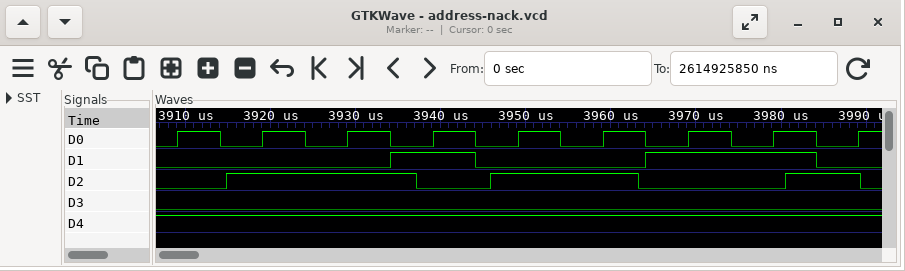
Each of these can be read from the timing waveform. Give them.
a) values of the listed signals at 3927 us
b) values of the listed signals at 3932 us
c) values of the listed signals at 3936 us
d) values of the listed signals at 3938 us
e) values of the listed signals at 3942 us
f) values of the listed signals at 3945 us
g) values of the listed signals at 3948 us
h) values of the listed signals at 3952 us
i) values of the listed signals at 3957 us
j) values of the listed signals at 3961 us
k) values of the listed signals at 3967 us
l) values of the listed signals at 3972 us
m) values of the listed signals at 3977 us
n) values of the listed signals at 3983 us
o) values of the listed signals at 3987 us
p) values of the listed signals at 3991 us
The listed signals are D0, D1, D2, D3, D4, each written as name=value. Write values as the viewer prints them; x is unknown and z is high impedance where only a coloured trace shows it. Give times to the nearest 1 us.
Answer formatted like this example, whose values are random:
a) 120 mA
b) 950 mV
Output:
a) D0=0, D1=0, D2=1, D3=0, D4=1
b) D0=1, D1=0, D2=1, D3=0, D4=1
c) D0=0, D1=1, D2=1, D3=0, D4=1
d) D0=0, D1=1, D2=0, D3=0, D4=1
e) D0=1, D1=1, D2=0, D3=0, D4=1
f) D0=0, D1=0, D2=0, D3=0, D4=1
g) D0=0, D1=0, D2=1, D3=0, D4=1
h) D0=1, D1=0, D2=1, D3=0, D4=1
i) D0=0, D1=0, D2=1, D3=0, D4=1
j) D0=1, D1=0, D2=1, D3=0, D4=1
k) D0=0, D1=1, D2=0, D3=0, D4=1
l) D0=1, D1=1, D2=0, D3=0, D4=1
m) D0=0, D1=1, D2=0, D3=0, D4=1
n) D0=1, D1=1, D2=1, D3=0, D4=1
o) D0=0, D1=0, D2=1, D3=0, D4=1
p) D0=1, D1=0, D2=0, D3=0, D4=1
